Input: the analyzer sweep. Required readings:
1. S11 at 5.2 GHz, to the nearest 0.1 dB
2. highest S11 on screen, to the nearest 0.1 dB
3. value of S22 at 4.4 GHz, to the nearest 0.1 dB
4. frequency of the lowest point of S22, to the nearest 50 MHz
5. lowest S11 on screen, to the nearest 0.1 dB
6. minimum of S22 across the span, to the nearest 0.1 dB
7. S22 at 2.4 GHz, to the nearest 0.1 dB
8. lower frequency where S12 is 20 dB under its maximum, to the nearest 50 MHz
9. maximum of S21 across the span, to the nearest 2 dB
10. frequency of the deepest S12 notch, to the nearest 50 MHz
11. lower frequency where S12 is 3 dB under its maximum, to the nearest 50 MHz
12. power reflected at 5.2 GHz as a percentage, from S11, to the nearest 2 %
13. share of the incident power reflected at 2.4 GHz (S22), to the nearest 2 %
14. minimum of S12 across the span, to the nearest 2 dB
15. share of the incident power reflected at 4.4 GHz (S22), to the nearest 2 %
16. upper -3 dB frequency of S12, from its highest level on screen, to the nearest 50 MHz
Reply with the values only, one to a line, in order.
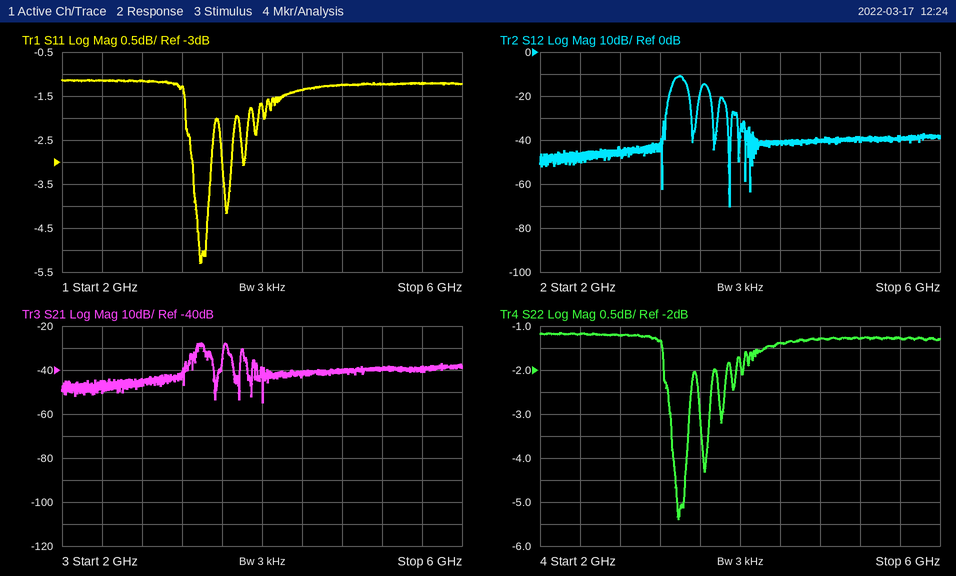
-1.2 dB
-1.1 dB
-1.4 dB
3.40 GHz
-5.3 dB
-5.4 dB
-1.2 dB
3.25 GHz
-28 dB
3.90 GHz
3.35 GHz
76 %
76 %
-70 dB
72 %
3.45 GHz
